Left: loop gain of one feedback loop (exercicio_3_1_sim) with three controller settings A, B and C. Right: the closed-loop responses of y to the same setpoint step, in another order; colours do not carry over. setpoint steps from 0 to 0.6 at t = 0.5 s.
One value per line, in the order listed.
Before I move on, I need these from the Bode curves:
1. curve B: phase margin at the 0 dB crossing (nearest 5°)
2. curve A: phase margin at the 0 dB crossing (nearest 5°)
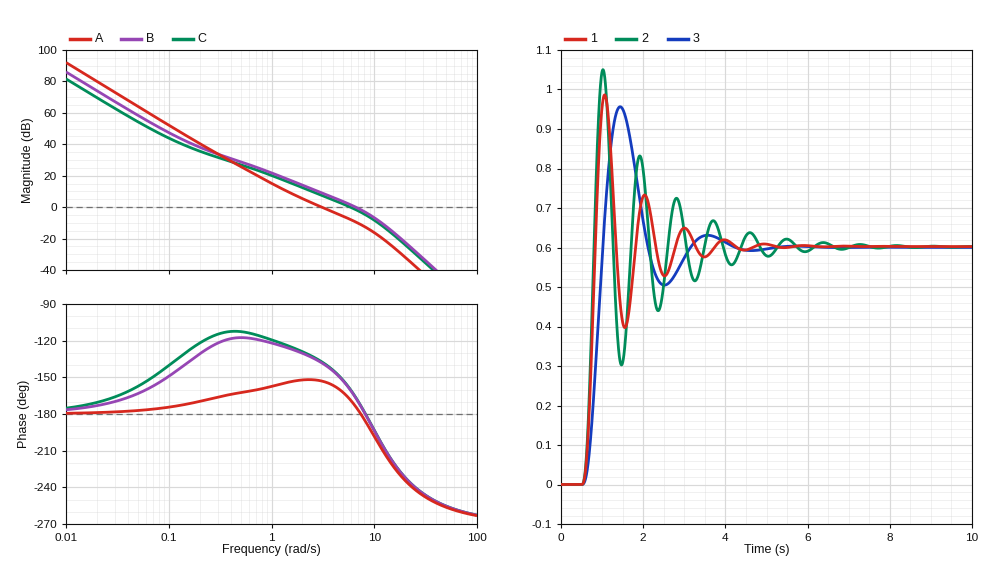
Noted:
15°
25°
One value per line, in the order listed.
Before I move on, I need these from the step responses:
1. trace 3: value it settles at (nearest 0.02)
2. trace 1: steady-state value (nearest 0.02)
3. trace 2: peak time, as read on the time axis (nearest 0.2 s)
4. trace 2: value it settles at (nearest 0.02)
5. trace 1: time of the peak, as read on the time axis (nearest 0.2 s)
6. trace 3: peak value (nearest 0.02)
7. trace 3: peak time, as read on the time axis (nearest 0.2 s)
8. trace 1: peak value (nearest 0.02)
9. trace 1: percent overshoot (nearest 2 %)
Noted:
0.60
0.60
1.0 s
0.60
1.0 s
0.96
1.4 s
0.98
64 %
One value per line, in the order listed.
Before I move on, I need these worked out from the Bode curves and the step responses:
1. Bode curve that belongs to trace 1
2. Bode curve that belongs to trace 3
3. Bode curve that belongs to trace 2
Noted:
C
A
B
